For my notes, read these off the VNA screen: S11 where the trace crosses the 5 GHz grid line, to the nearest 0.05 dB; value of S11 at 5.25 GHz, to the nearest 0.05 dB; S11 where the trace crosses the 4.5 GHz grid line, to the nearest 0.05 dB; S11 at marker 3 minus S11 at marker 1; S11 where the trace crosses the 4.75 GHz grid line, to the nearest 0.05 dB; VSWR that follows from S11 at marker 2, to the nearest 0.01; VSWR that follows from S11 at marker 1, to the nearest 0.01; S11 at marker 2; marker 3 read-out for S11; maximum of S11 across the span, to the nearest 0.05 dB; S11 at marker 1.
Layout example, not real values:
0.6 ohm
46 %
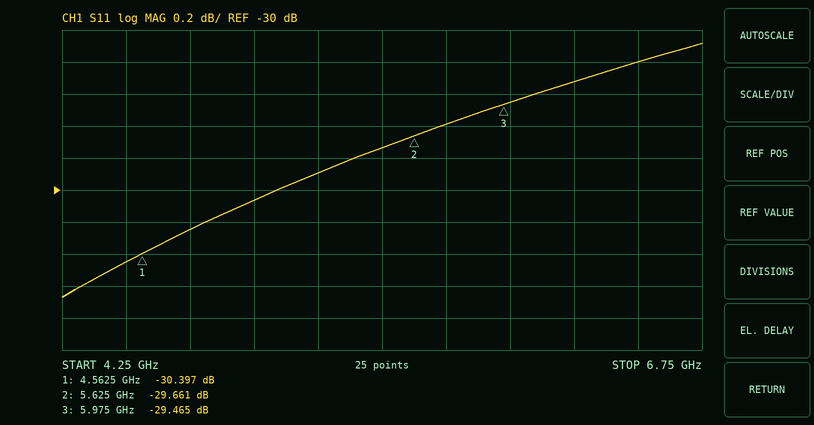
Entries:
-30.05 dB
-29.90 dB
-30.45 dB
0.932 dB
-30.25 dB
1.07
1.06
-29.661 dB
-29.465 dB
-29.10 dB
-30.397 dB
